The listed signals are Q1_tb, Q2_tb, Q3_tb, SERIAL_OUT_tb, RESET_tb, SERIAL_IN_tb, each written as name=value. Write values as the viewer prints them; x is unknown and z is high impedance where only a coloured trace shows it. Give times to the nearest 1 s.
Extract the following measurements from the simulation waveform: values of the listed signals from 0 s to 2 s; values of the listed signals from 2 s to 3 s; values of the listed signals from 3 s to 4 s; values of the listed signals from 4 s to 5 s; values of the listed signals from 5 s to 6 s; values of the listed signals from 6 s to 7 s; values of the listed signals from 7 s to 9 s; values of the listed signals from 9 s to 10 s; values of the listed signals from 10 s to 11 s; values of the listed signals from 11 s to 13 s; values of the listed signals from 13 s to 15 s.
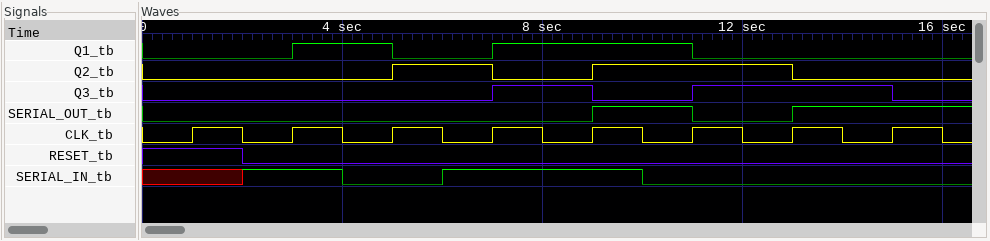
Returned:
Q1_tb=0, Q2_tb=0, Q3_tb=0, SERIAL_OUT_tb=0, RESET_tb=1, SERIAL_IN_tb=x
Q1_tb=0, Q2_tb=0, Q3_tb=0, SERIAL_OUT_tb=0, RESET_tb=0, SERIAL_IN_tb=1
Q1_tb=1, Q2_tb=0, Q3_tb=0, SERIAL_OUT_tb=0, RESET_tb=0, SERIAL_IN_tb=1
Q1_tb=1, Q2_tb=0, Q3_tb=0, SERIAL_OUT_tb=0, RESET_tb=0, SERIAL_IN_tb=0
Q1_tb=0, Q2_tb=1, Q3_tb=0, SERIAL_OUT_tb=0, RESET_tb=0, SERIAL_IN_tb=0
Q1_tb=0, Q2_tb=1, Q3_tb=0, SERIAL_OUT_tb=0, RESET_tb=0, SERIAL_IN_tb=1
Q1_tb=1, Q2_tb=0, Q3_tb=1, SERIAL_OUT_tb=0, RESET_tb=0, SERIAL_IN_tb=1
Q1_tb=1, Q2_tb=1, Q3_tb=0, SERIAL_OUT_tb=1, RESET_tb=0, SERIAL_IN_tb=1
Q1_tb=1, Q2_tb=1, Q3_tb=0, SERIAL_OUT_tb=1, RESET_tb=0, SERIAL_IN_tb=0
Q1_tb=0, Q2_tb=1, Q3_tb=1, SERIAL_OUT_tb=0, RESET_tb=0, SERIAL_IN_tb=0
Q1_tb=0, Q2_tb=0, Q3_tb=1, SERIAL_OUT_tb=1, RESET_tb=0, SERIAL_IN_tb=0
